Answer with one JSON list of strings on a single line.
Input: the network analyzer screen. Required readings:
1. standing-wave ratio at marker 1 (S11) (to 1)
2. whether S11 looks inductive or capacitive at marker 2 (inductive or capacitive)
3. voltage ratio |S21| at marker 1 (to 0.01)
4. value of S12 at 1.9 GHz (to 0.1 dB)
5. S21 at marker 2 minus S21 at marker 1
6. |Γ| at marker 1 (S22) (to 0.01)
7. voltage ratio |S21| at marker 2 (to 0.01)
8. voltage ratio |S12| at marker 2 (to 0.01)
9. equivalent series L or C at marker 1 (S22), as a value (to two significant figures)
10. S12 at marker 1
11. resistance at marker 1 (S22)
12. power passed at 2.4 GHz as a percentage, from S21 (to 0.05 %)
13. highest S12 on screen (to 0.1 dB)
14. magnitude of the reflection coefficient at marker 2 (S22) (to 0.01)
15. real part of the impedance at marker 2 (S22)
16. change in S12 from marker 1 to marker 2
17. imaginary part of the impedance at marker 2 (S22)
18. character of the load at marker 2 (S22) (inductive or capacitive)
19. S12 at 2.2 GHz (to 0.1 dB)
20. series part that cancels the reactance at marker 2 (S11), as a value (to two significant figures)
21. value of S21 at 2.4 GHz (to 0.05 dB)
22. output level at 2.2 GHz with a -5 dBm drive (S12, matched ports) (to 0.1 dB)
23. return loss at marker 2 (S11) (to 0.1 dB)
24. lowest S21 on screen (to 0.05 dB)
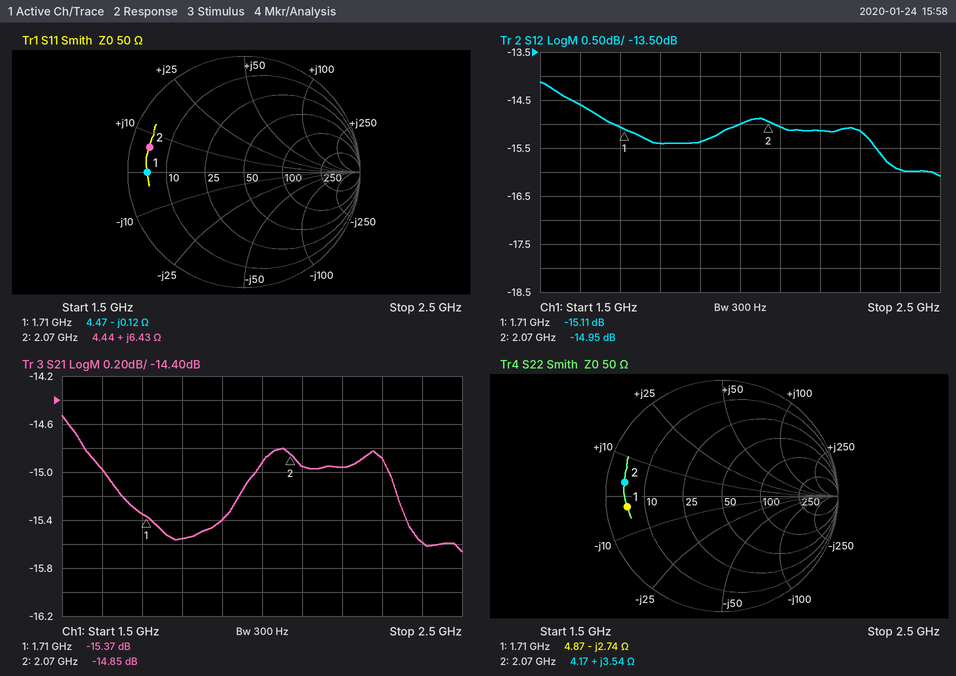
["11", "inductive", "0.17", "-15.4 dB", "0.52 dB", "0.82", "0.18", "0.18", "34 pF", "-15.11 dB", "4.87 Ω", "2.75 %", "-14.1 dB", "0.85", "4.17 Ω", "0.16 dB", "+3.54 Ω", "inductive", "-15.1 dB", "12 pF", "-15.60 dB", "-20.1 dBm", "1.5 dB", "-15.65 dB"]
